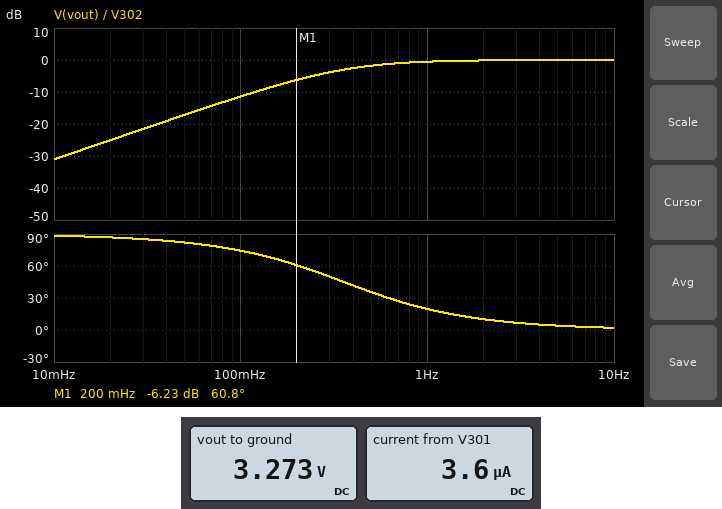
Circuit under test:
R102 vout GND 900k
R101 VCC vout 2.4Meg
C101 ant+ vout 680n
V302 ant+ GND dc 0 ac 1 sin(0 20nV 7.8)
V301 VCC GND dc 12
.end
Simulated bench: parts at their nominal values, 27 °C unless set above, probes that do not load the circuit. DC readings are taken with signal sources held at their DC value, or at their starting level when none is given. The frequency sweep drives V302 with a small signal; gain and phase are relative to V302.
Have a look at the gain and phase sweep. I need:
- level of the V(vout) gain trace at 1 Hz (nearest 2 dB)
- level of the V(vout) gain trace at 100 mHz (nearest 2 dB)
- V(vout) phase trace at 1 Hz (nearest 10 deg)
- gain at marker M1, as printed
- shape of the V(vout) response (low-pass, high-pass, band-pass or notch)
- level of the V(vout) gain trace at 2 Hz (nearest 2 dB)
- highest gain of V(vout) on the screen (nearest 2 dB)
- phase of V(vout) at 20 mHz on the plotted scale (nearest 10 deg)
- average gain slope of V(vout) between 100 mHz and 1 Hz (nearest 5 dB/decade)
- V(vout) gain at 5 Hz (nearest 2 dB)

0 dB
-12 dB
20 deg
-6.23 dB
high-pass
0 dB
0 dB
90 deg
10 dB/decade
0 dB
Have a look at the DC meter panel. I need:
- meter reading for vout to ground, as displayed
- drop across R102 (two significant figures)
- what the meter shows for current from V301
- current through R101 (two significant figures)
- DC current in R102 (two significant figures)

3.273 V
3.3 V
3.6 µA
3.6 µA
3.6 µA
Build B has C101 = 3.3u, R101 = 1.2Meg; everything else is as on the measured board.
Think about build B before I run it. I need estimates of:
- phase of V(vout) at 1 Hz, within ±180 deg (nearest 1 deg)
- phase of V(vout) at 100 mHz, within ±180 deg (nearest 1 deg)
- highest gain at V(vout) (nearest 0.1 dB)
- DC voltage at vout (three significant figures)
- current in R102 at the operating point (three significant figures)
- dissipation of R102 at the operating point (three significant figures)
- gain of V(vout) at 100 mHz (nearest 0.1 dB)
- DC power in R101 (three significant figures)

5 deg
43 deg
0 dB
5.14 V
5.71 µA
29.4 µW
-2.7 dB
39.2 µW
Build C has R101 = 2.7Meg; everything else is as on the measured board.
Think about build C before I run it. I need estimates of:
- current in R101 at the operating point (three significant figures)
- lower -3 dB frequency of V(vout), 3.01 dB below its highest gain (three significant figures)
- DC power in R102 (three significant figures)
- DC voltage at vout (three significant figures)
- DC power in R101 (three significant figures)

3.33 µA
347 mHz
10.0 µW
3.00 V
30.0 µW
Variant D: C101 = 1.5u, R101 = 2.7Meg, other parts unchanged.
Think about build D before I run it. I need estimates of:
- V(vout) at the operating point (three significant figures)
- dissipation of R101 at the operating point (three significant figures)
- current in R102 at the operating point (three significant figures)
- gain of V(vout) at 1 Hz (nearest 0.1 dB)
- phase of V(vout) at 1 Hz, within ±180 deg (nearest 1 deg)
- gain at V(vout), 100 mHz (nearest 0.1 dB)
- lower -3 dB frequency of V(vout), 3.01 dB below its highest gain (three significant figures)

3.00 V
30.0 µW
3.33 µA
-0.1 dB
9 deg
-5.4 dB
157 mHz
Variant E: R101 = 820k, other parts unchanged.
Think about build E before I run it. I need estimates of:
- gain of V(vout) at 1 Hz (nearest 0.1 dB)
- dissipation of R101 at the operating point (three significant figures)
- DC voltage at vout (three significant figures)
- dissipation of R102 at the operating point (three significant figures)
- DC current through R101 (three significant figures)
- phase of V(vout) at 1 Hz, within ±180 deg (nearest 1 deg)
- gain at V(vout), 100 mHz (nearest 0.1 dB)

-1.1 dB
39.9 µW
6.28 V
43.8 µW
6.98 µA
29 deg
-14.9 dB
